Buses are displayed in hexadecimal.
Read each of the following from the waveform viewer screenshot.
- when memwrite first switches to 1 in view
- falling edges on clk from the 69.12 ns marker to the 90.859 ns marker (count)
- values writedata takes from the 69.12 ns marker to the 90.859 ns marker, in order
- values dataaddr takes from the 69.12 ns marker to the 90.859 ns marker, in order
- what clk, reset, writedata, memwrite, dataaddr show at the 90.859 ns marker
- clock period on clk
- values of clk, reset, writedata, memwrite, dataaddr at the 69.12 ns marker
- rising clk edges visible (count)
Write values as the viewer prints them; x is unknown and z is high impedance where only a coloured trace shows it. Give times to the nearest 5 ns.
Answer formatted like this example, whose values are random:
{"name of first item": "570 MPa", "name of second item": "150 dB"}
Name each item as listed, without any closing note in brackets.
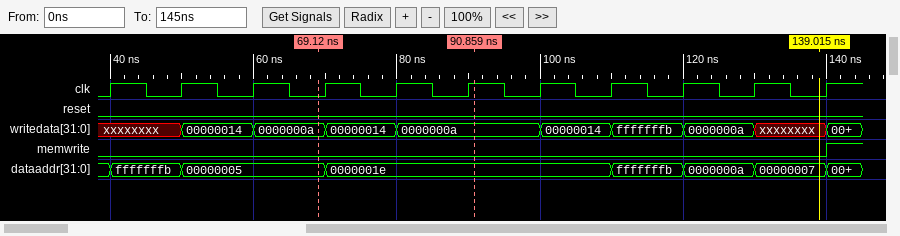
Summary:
{"when memwrite first switches to 1 in view": "140 ns", "falling edges on clk from the 69.12 ns marker to the 90.859 ns marker": "2", "values writedata takes from the 69.12 ns marker to the 90.859 ns marker, in order": "0000000a, 00000014, 0000000a", "values dataaddr takes from the 69.12 ns marker to the 90.859 ns marker, in order": "00000005, 0000001e", "what clk, reset, writedata, memwrite, dataaddr show at the 90.859 ns marker": "clk=1, reset=0, writedata=0000000a, memwrite=0, dataaddr=0000001e", "clock period on clk": "10 ns", "values of clk, reset, writedata, memwrite, dataaddr at the 69.12 ns marker": "clk=0, reset=0, writedata=0000000a, memwrite=0, dataaddr=00000005", "rising clk edges visible": "11"}
